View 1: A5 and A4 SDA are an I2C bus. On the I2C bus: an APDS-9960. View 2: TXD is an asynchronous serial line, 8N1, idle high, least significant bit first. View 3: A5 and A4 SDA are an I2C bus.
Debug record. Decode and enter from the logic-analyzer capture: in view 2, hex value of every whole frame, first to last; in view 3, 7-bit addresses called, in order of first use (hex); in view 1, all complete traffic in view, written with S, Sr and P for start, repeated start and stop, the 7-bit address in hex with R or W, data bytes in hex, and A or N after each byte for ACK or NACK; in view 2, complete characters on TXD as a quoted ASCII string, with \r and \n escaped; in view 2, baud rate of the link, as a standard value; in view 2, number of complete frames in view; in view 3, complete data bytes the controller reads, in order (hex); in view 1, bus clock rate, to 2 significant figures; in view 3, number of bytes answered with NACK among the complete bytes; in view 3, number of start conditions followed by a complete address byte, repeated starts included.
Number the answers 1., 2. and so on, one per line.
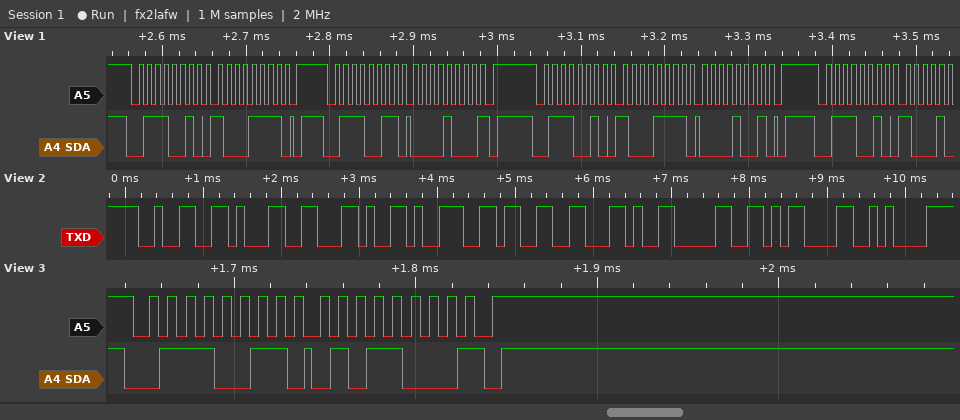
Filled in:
1. 32 31 2C 39 33 2C 30 0D 0A
2. 0x39
3. S 39W A 8F A P S 39R A 08 N P S 39W A 8F A 09 A P S 39W A
4. "21,93,0\r\n"
5. 9600 baud
6. 9
7. 58
8. 100 kHz
9. 1
10. 1
